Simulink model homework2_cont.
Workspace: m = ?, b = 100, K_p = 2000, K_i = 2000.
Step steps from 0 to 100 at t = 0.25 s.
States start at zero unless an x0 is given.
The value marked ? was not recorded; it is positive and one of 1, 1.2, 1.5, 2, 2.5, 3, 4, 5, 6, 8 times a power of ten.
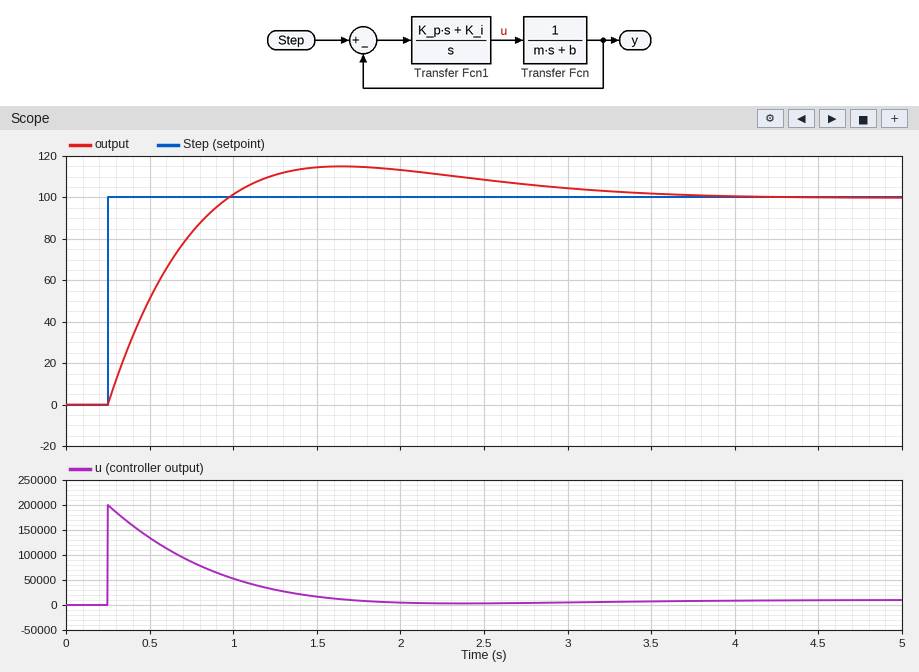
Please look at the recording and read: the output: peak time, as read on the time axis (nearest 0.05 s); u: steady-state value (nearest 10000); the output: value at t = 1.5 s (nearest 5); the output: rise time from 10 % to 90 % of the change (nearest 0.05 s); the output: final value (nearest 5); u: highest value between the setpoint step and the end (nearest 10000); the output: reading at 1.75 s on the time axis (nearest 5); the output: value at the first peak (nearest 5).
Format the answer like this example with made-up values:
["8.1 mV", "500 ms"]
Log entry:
["1.65 s", "10000", "115", "0.55 s", "100", "200000", "115", "115"]
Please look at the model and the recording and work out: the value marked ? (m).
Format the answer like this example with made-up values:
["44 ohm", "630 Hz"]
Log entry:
["800"]
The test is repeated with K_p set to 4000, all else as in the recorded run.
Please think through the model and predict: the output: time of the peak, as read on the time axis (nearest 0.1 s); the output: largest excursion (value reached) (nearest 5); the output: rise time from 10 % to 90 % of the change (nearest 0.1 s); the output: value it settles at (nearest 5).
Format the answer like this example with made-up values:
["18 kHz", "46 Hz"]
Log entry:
["1.4 s", "105", "0.4 s", "100"]
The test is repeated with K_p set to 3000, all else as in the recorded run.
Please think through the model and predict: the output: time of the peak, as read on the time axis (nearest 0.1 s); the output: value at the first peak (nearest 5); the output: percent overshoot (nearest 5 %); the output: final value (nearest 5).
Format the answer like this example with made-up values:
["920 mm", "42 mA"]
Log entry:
["1.5 s", "110", "10 %", "100"]
